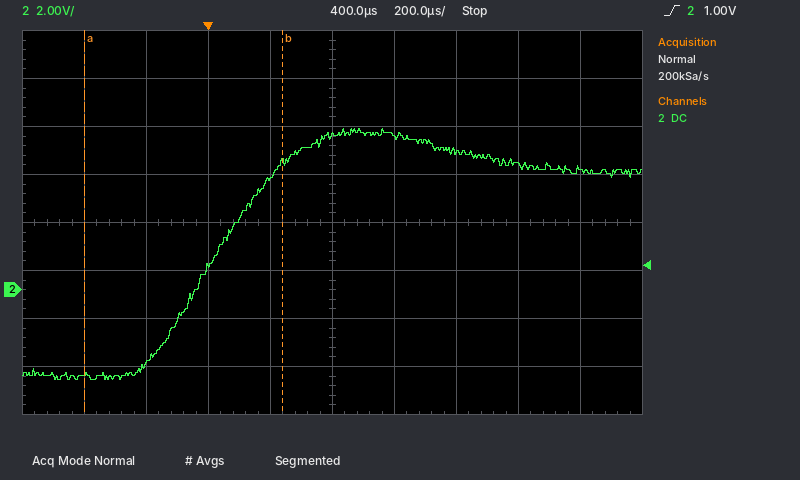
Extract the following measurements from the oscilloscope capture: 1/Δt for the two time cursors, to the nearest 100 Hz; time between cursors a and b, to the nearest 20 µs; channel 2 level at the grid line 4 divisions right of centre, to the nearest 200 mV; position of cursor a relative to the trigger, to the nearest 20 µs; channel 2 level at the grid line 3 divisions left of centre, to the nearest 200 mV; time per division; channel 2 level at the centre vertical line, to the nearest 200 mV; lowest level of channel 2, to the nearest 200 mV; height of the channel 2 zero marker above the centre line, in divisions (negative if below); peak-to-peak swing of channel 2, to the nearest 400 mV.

1.6 kHz
640 µs
5.0 V
-400 µs
-3.2 V
200 µs
6.4 V
-3.8 V
-1.4 div
10.4 V
